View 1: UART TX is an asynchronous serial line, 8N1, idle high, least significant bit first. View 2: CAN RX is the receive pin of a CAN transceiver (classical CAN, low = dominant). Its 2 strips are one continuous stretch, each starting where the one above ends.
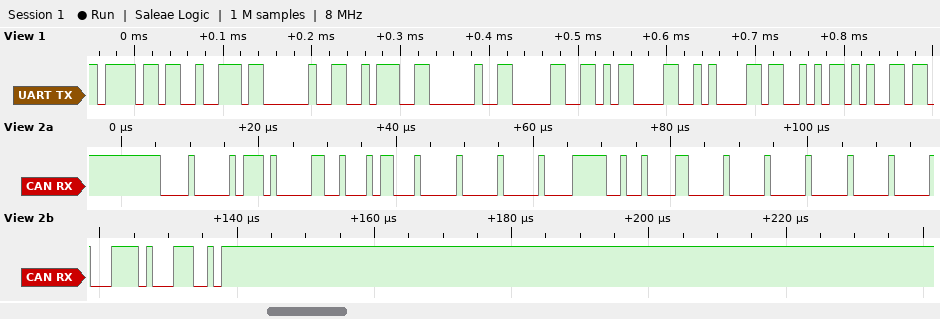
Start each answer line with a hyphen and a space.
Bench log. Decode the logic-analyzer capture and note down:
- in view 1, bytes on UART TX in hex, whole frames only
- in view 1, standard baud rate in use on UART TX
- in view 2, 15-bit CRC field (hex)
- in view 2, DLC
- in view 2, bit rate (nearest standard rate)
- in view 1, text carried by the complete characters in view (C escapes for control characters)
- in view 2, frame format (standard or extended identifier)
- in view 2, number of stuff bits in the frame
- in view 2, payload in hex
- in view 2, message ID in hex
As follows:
- 6F 72 20 3A 20 30 0D 0A 53 65
- 115200 baud
- 0x3D1C
- 8
- 1000 kbit/s
- "or : 0\r\nSe"
- extended
- 12
- 00 00 FA 43 00 00 00 00
- 0x0205048B
